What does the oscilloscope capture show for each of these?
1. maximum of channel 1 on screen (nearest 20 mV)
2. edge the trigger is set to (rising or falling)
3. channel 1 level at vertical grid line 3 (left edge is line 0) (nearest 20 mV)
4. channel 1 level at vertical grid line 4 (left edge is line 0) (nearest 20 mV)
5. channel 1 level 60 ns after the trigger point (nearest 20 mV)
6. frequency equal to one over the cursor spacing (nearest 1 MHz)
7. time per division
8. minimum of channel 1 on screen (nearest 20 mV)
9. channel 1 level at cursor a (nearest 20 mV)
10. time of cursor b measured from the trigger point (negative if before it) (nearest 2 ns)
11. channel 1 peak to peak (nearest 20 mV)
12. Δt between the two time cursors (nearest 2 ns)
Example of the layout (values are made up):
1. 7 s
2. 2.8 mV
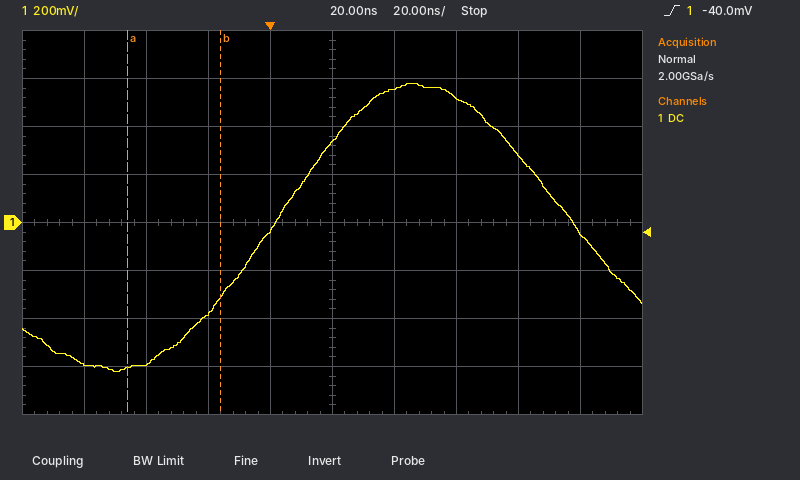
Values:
1. 580 mV
2. rising
3. -380 mV
4. -40 mV
5. 520 mV
6. 33 MHz
7. 20 ns
8. -620 mV
9. -600 mV
10. -16 ns
11. 1.20 V
12. 30 ns
